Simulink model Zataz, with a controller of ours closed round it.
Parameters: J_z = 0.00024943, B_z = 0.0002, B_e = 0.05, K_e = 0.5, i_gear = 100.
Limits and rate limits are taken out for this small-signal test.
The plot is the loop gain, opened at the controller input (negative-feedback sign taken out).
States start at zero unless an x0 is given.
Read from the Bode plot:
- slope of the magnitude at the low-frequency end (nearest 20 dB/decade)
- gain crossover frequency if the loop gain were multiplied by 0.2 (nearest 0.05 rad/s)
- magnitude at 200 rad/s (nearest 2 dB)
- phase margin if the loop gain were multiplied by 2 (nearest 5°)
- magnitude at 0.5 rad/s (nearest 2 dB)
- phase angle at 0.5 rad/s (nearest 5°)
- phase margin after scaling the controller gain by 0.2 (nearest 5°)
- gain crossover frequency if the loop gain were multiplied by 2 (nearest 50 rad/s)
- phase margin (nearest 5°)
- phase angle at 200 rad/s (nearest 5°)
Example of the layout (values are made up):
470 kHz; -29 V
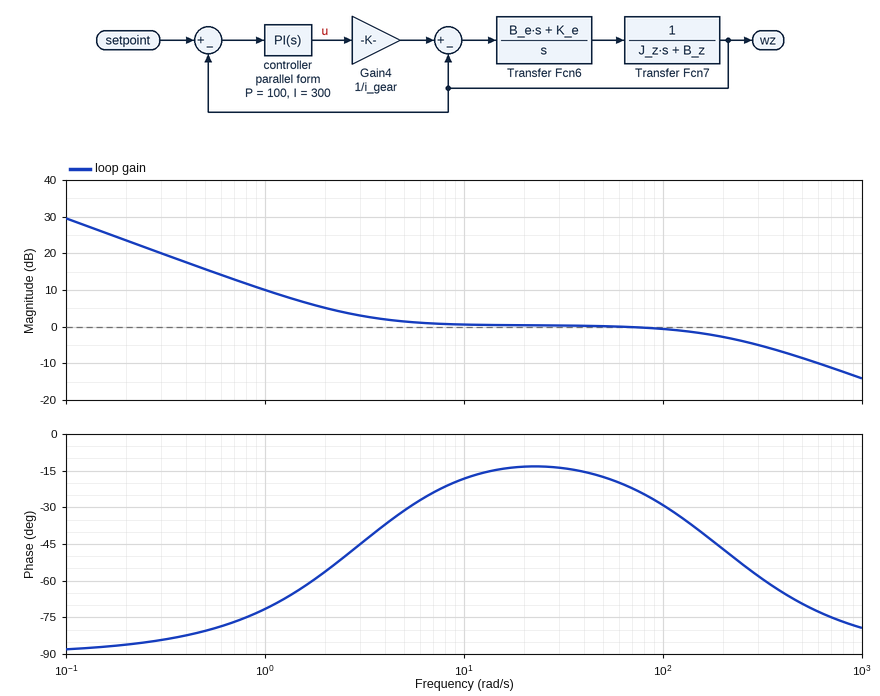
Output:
-20 dB/decade; 0.60 rad/s; -2 dB; 120°; 16 dB; -80°; 100°; 350 rad/s; 160°; -45°
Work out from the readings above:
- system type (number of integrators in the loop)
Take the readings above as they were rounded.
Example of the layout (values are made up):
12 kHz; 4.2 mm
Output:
1
